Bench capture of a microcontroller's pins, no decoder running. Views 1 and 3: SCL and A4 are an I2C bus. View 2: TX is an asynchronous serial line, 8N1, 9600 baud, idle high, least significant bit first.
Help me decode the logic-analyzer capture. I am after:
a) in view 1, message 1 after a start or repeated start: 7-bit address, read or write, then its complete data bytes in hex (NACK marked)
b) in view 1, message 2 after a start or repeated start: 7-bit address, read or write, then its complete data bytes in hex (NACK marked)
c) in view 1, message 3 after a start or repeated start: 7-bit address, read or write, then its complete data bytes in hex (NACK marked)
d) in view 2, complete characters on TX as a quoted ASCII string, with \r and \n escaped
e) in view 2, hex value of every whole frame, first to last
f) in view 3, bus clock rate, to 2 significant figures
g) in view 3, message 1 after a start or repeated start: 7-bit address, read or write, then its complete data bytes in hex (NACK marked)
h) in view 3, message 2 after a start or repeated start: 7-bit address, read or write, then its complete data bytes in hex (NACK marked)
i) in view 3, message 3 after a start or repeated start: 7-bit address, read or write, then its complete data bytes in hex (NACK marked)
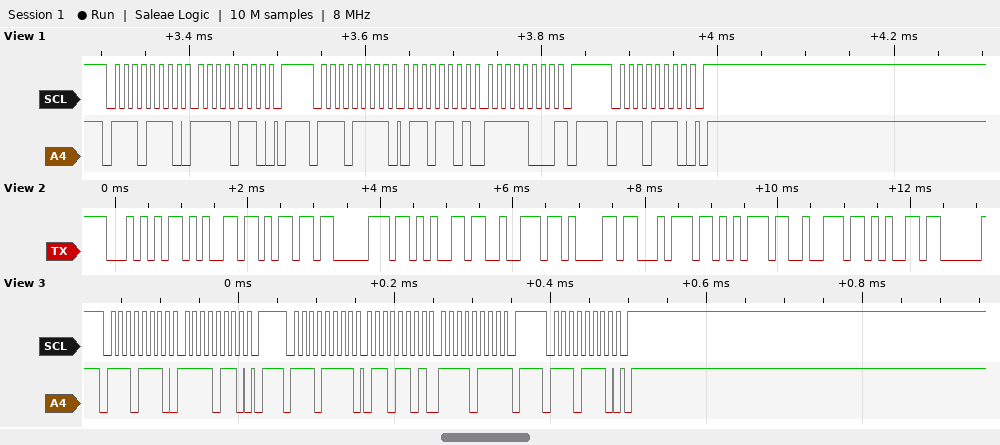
0x77 write: F6
0x77 read: 6D F8 NACK
0x77 write
"Temperature"
54 65 6D 70 65 72 61 74 75 72 65
100 kHz
0x77 write: F6
0x77 read: 6D F7 NACK
0x77 write
